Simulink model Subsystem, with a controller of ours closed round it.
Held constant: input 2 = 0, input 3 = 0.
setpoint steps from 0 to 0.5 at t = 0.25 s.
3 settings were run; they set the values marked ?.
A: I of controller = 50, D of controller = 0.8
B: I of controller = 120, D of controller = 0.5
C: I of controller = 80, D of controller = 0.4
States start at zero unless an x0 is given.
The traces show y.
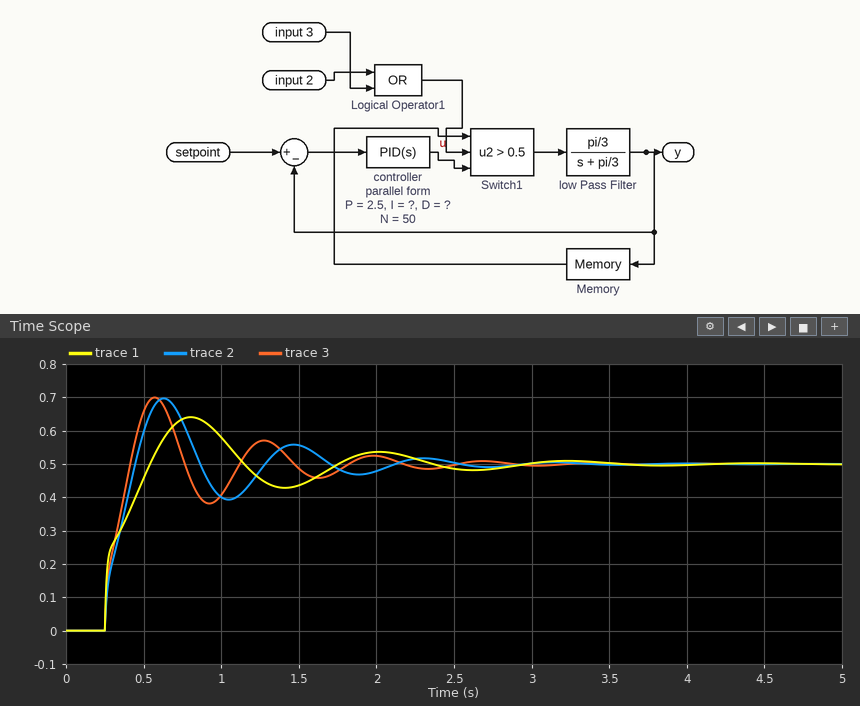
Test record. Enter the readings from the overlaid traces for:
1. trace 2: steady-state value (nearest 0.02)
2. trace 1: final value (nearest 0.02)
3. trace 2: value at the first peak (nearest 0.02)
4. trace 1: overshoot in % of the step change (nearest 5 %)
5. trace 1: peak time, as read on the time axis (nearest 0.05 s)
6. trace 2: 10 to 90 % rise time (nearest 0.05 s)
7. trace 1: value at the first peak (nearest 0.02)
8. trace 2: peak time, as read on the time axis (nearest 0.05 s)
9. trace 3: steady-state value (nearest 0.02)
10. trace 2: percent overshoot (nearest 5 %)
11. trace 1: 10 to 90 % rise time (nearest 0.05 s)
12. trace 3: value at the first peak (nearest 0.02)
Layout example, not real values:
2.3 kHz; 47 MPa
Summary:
0.50; 0.50; 0.70; 30 %; 0.80 s; 0.15 s; 0.64; 0.65 s; 0.50; 40 %; 0.25 s; 0.70
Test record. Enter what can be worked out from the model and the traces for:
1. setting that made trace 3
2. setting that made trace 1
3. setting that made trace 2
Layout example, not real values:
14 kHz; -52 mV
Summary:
B; A; C
